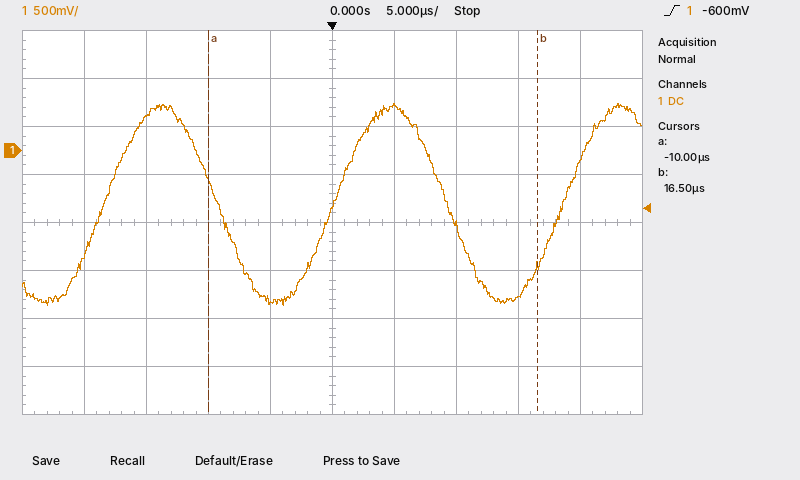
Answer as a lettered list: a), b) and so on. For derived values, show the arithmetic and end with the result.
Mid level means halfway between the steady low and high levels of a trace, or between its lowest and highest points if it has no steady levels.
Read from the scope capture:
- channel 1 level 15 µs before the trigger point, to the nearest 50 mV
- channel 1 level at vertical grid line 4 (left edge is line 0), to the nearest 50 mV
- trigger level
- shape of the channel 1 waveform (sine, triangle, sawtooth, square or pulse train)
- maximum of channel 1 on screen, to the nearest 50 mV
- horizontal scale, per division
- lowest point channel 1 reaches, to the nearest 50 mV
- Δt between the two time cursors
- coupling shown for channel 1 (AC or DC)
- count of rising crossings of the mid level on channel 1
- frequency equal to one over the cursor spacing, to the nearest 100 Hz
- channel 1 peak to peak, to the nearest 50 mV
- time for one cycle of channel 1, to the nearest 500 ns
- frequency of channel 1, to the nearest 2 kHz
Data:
a) 350 mV
b) -1.55 V
c) -600 mV
d) sine
e) 500 mV
f) 5 µs
g) -1.60 V
h) 16.5 µs − (-10 µs) = 26.5 µs
i) DC
j) 3
k) 1 / 26.5 µs ≈ 37.7 kHz
l) 500 mV − (-1.60 V) = 2.10 V
m) 18.5 µs
n) 1 / 18.5 µs ≈ 54 kHz
